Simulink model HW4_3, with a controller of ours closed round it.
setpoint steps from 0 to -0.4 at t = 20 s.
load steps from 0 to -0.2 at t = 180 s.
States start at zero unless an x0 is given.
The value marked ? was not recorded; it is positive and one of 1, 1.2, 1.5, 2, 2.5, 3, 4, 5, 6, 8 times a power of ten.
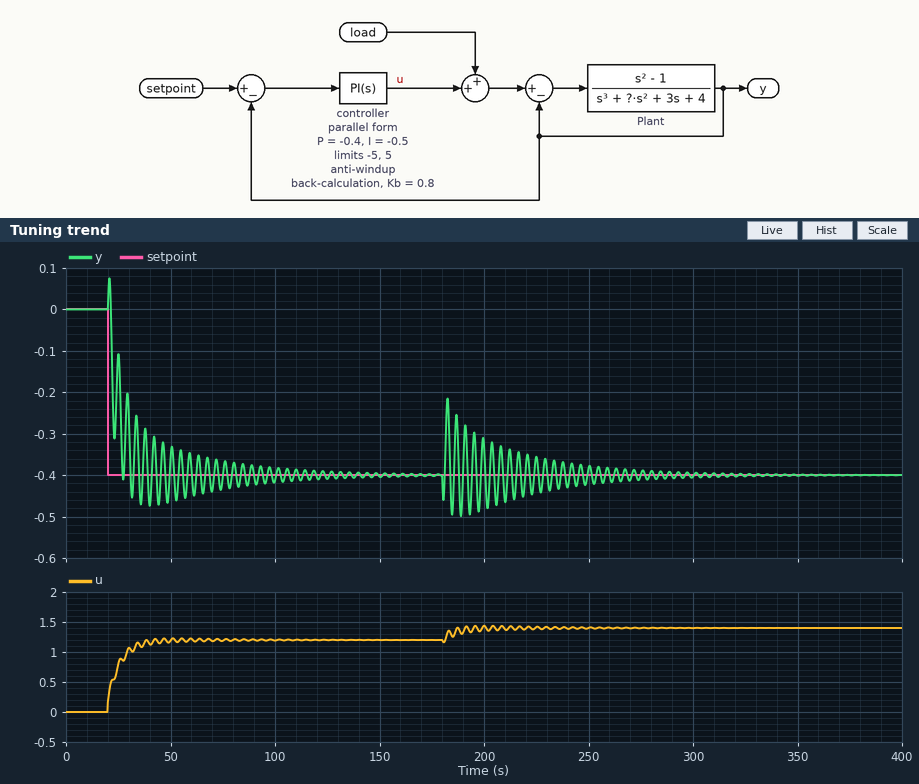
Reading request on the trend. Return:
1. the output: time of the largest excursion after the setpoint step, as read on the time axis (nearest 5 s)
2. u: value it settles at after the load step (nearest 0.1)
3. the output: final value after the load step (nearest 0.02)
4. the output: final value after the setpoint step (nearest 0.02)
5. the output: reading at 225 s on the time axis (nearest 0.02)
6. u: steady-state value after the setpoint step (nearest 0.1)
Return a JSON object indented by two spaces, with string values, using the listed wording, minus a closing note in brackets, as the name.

{
  "the output: time of the largest excursion after the setpoint step, as read on the time axis": "40 s",
  "u: value it settles at after the load step": "1.4",
  "the output: final value after the load step": "-0.40",
  "the output: final value after the setpoint step": "-0.40",
  "the output: reading at 225 s on the time axis": "-0.36",
  "u: steady-state value after the setpoint step": "1.2"
}
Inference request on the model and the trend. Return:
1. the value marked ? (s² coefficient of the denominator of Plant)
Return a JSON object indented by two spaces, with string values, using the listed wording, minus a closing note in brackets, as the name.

{
  "the value marked ?": "1"
}
